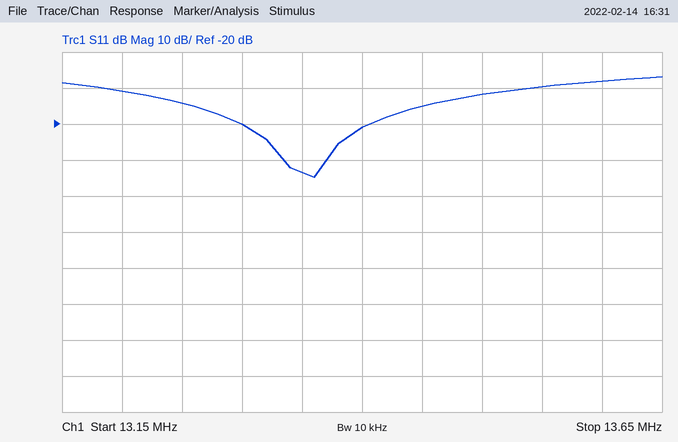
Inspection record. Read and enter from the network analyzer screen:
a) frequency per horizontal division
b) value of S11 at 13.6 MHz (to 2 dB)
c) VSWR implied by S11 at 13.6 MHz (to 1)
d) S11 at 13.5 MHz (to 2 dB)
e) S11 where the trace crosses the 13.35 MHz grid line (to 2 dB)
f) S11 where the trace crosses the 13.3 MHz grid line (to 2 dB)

50 kHz
-8 dB
2
-12 dB
-34 dB
-20 dB
